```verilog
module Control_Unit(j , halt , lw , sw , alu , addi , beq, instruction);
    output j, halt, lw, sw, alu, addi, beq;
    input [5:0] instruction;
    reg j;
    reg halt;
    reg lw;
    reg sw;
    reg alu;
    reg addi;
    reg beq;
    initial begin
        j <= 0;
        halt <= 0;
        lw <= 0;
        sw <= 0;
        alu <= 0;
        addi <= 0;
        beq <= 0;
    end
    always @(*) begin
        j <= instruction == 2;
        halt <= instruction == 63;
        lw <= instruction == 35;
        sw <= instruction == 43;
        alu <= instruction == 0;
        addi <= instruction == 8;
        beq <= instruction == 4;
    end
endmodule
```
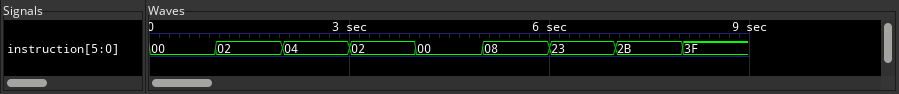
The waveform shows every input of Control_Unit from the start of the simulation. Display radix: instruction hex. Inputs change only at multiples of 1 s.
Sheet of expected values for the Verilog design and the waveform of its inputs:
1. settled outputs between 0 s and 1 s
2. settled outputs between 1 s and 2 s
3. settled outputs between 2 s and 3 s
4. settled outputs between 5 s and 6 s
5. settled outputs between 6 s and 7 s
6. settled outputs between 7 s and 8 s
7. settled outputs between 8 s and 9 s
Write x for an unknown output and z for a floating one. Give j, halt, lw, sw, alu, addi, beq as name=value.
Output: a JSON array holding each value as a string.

["j=0, halt=0, lw=0, sw=0, alu=1, addi=0, beq=0", "j=1, halt=0, lw=0, sw=0, alu=0, addi=0, beq=0", "j=0, halt=0, lw=0, sw=0, alu=0, addi=0, beq=1", "j=0, halt=0, lw=0, sw=0, alu=0, addi=1, beq=0", "j=0, halt=0, lw=1, sw=0, alu=0, addi=0, beq=0", "j=0, halt=0, lw=0, sw=1, alu=0, addi=0, beq=0", "j=0, halt=1, lw=0, sw=0, alu=0, addi=0, beq=0"]
